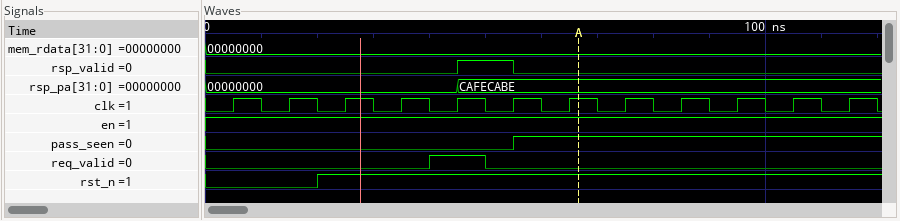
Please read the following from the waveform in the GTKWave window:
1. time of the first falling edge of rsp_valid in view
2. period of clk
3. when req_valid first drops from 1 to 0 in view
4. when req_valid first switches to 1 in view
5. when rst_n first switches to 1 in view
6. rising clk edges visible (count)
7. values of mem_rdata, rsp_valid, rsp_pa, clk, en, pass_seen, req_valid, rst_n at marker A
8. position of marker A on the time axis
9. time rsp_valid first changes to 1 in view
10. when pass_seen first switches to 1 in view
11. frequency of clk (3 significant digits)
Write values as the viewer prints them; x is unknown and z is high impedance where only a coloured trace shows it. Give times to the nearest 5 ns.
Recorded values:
55 ns
10 ns
50 ns
40 ns
20 ns
12
mem_rdata=00000000, rsp_valid=0, rsp_pa=CAFECABE, clk=1, en=1, pass_seen=1, req_valid=0, rst_n=1
65 ns
45 ns
55 ns
100 MHz
